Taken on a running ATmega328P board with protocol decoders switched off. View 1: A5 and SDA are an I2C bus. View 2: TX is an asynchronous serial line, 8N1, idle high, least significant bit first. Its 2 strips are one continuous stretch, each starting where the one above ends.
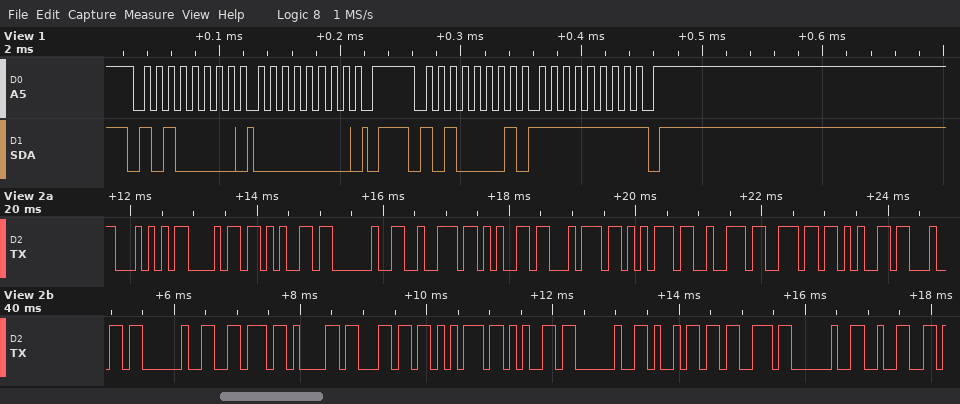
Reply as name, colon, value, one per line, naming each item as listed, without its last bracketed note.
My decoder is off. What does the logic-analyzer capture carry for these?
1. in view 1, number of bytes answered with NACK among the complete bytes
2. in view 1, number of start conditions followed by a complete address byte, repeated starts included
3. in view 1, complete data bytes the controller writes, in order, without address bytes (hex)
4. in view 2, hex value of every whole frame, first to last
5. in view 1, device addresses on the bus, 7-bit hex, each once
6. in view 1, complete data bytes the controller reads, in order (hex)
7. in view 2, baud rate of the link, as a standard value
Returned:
in view 1, number of bytes answered with NACK among the complete bytes: 1
in view 1, number of start conditions followed by a complete address byte, repeated starts included: 2
in view 1, complete data bytes the controller writes, in order, without address bytes: 00
in view 2, hex value of every whole frame, first to last: 54 68 65 20 72 65 74 75 72 6E 65 64 20 76 61 6C 75 65 20 69 73 20 32
in view 1, device addresses on the bus, 7-bit hex, each once: 0x50
in view 1, complete data bytes the controller reads, in order: FF
in view 2, baud rate of the link, as a standard value: 9600 baud
